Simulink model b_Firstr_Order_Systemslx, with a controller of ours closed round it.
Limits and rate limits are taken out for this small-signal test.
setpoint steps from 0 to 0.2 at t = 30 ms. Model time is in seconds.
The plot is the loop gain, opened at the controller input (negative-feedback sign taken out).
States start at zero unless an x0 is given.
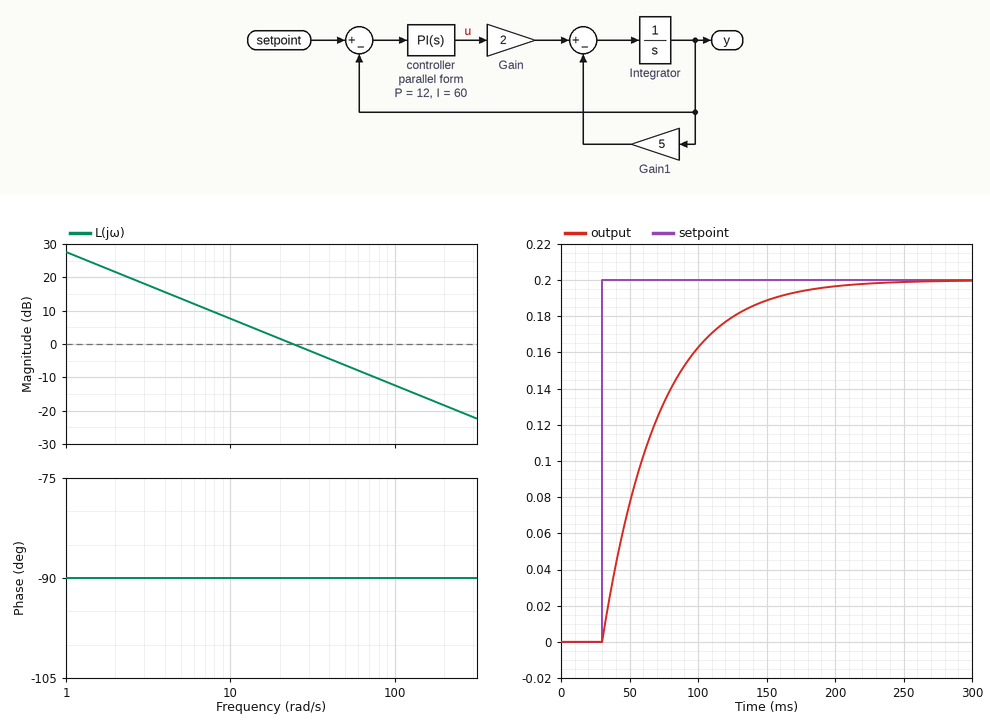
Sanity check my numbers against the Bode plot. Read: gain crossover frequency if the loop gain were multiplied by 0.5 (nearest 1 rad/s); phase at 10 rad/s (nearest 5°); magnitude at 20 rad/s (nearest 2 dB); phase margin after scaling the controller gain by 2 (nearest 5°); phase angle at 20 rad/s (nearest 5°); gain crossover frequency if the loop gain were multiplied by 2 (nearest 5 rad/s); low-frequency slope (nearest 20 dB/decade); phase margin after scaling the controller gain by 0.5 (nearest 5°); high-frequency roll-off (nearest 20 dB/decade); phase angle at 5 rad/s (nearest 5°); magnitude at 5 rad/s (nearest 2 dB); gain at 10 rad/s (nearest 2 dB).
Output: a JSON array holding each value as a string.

["12 rad/s", "-90°", "2 dB", "90°", "-90°", "50 rad/s", "-20 dB/decade", "90°", "-20 dB/decade", "-90°", "14 dB", "8 dB"]
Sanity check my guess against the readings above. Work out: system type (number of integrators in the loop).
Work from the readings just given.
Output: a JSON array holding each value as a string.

["1"]
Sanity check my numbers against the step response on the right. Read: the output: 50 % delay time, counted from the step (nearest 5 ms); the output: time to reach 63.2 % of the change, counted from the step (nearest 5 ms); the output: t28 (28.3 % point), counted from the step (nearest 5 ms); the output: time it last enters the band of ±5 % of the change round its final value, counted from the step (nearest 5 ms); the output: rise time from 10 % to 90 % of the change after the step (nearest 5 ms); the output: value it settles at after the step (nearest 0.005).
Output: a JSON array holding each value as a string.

["30 ms", "40 ms", "15 ms", "125 ms", "90 ms", "0.200"]
